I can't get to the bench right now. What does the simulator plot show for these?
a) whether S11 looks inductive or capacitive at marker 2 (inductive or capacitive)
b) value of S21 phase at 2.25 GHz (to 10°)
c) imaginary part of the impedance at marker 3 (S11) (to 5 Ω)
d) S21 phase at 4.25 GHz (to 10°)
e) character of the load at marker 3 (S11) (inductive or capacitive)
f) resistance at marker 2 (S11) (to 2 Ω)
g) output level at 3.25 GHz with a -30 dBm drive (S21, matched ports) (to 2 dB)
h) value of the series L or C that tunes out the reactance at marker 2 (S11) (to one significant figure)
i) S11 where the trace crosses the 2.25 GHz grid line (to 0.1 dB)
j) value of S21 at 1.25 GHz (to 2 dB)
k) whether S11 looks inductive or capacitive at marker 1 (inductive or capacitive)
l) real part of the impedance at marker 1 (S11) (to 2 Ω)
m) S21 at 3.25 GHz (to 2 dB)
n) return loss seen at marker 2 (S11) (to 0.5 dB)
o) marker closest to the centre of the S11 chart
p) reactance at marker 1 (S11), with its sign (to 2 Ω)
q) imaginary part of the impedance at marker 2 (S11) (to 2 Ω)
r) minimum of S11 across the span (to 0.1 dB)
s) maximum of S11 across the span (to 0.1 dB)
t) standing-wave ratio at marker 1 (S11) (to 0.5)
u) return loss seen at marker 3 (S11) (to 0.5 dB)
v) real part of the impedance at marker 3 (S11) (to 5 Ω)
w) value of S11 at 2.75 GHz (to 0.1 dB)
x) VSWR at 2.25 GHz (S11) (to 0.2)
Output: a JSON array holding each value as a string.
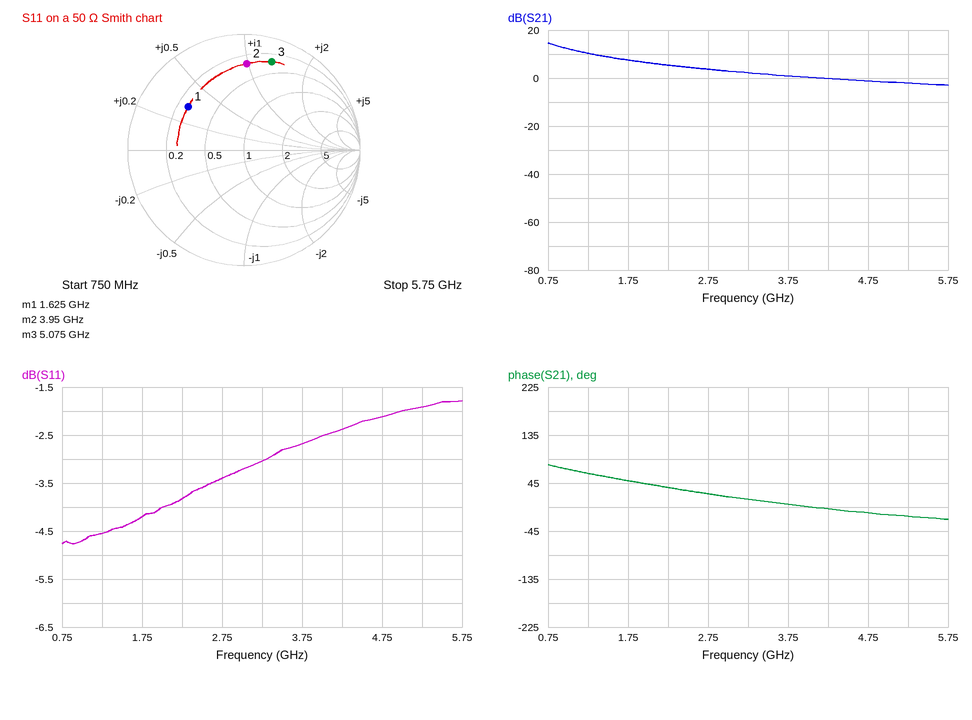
["inductive", "40°", "+65 Ω", "0°", "inductive", "14 Ω", "-28 dBm", "800 fF", "-3.8 dB", "10 dB", "inductive", "14 Ω", "2 dB", "2.5 dB", "marker 1", "+16 Ω", "+50 Ω", "-4.8 dB", "-1.8 dB", "4.0", "2.0 dB", "15 Ω", "-3.4 dB", "4.6"]
